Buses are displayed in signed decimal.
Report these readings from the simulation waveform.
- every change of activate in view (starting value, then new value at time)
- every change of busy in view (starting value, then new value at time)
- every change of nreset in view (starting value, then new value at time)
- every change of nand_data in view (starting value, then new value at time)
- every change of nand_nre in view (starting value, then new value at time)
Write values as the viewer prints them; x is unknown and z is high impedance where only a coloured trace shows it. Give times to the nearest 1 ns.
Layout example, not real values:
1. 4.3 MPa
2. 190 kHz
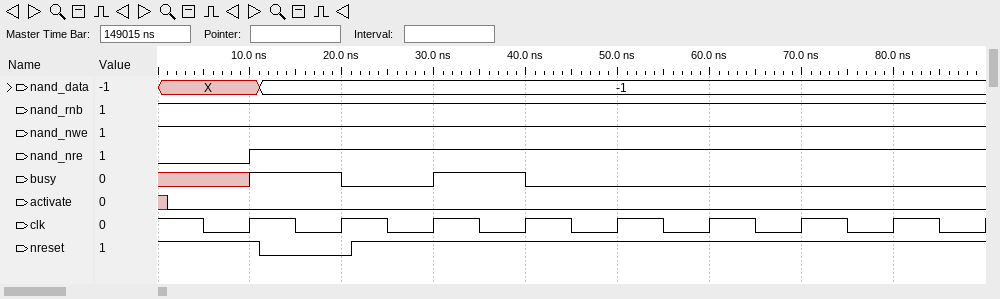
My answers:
1. x, 0 at 1 ns
2. x, 1 at 10 ns, 0 at 20 ns, 1 at 30 ns, 0 at 40 ns
3. 1, 0 at 11 ns, 1 at 21 ns
4. X, -1 at 11 ns
5. 0, 1 at 10 ns
